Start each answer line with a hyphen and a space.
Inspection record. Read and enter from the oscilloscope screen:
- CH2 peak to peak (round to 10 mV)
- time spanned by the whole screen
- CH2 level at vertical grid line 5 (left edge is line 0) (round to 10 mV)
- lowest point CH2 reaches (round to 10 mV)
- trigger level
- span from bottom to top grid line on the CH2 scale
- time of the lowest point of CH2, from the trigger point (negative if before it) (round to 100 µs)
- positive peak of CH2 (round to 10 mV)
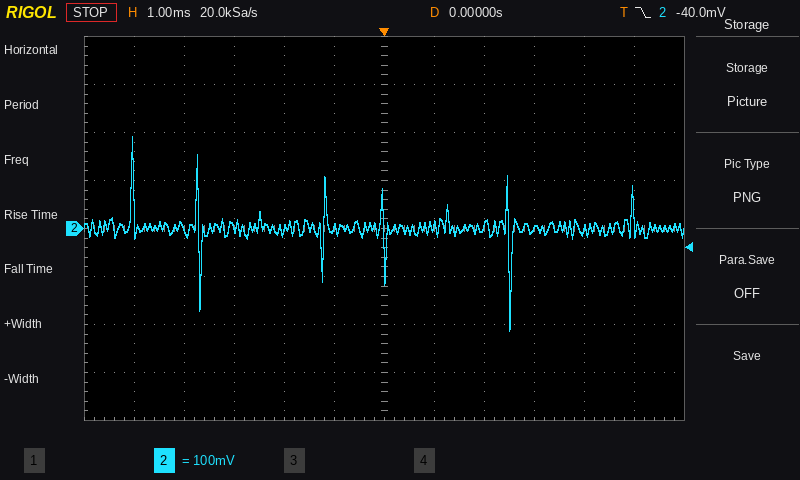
- 400 mV
- 12 ms
- 0 mV
- -210 mV
- -40.0 mV
- 800 mV
- +2.5 ms
- 190 mV
